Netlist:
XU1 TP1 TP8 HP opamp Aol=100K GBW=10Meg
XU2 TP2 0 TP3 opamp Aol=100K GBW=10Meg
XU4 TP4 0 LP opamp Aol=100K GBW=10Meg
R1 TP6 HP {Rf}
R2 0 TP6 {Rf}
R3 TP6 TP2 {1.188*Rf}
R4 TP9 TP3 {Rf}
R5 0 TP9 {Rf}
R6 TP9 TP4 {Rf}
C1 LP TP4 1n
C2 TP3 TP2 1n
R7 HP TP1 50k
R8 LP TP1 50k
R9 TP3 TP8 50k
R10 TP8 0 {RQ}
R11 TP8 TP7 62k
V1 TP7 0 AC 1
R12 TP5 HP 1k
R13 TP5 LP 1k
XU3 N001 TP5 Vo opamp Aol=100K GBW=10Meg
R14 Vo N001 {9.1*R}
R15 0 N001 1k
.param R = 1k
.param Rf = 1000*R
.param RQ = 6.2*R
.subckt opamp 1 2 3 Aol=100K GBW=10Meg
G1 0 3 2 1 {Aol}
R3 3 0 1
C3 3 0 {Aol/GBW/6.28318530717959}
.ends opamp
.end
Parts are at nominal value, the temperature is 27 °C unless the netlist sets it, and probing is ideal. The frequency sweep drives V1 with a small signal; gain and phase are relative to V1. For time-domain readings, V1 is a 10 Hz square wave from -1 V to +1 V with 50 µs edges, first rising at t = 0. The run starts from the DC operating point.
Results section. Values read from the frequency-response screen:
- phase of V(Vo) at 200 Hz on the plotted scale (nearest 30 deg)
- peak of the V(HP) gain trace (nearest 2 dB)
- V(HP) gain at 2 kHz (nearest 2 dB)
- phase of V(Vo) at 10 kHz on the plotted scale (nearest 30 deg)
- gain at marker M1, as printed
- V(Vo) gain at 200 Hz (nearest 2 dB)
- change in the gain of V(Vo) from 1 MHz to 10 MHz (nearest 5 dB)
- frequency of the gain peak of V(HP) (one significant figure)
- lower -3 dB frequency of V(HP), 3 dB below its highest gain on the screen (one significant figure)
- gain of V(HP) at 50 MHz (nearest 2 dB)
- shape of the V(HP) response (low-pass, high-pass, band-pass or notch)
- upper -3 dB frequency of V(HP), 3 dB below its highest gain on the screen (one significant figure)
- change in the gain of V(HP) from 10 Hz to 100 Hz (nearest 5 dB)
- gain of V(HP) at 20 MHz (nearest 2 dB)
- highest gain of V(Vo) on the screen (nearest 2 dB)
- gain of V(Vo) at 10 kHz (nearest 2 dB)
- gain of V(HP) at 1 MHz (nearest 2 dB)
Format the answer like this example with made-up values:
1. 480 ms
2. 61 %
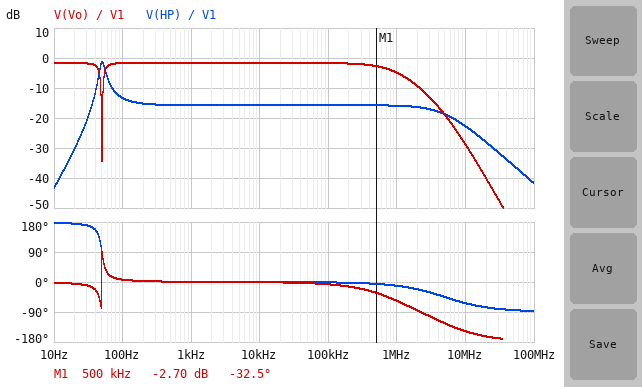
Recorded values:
1. 0 deg
2. -2 dB
3. -16 dB
4. 0 deg
5. -2.70 dB
6. -2 dB
7. -25 dB
8. 50 Hz
9. 50 Hz
10. -36 dB
11. band-pass
12. 60 Hz
13. 30 dB
14. -28 dB
15. -2 dB
16. -2 dB
17. -16 dB
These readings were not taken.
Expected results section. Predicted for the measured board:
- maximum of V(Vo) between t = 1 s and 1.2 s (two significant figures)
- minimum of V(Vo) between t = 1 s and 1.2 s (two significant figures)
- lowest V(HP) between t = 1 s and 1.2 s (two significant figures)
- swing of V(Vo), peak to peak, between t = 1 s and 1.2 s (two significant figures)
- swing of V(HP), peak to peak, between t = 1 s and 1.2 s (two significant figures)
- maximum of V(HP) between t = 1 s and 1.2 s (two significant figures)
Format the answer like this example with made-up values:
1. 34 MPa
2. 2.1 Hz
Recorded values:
1. 1.1 V
2. -1.1 V
3. -420 mV
4. 2.2 V
5. 840 mV
6. 420 mV
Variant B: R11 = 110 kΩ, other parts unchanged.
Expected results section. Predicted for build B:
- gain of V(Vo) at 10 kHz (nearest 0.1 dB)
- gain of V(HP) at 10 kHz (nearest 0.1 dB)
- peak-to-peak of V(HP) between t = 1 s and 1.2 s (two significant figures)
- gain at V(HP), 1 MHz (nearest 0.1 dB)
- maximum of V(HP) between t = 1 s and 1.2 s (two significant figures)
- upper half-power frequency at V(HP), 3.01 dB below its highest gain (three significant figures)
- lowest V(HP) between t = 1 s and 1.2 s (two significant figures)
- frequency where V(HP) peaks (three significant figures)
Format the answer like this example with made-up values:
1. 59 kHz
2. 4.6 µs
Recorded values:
1. -6.3 dB
2. -20.4 dB
3. 480 mV
4. -20.6 dB
5. 240 mV
6. 56.5 Hz
7. -240 mV
8. 50.5 Hz
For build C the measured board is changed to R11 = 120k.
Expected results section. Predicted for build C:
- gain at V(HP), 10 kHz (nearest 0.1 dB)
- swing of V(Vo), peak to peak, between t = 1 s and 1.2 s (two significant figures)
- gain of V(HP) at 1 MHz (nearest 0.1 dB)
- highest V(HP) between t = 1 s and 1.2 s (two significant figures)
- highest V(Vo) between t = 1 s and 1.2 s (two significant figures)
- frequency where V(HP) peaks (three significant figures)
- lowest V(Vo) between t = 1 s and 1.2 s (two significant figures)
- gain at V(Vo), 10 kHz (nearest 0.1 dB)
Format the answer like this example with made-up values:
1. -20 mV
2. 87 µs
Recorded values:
1. -21.1 dB
2. 1.2 V
3. -21.3 dB
4. 220 mV
5. 580 mV
6. 50.5 Hz
7. -580 mV
8. -7.1 dB
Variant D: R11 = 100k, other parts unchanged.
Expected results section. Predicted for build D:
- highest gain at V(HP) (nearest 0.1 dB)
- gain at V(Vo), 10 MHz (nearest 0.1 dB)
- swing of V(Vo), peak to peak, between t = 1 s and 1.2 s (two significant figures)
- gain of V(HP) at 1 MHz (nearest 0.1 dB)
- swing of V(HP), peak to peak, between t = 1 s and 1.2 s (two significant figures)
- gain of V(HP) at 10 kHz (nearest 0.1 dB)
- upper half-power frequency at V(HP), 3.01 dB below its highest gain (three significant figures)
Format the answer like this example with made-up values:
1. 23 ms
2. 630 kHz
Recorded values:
1. -5.5 dB
2. -32.7 dB
3. 1.4 V
4. -19.8 dB
5. 530 mV
6. -19.6 dB
7. 56.5 Hz
